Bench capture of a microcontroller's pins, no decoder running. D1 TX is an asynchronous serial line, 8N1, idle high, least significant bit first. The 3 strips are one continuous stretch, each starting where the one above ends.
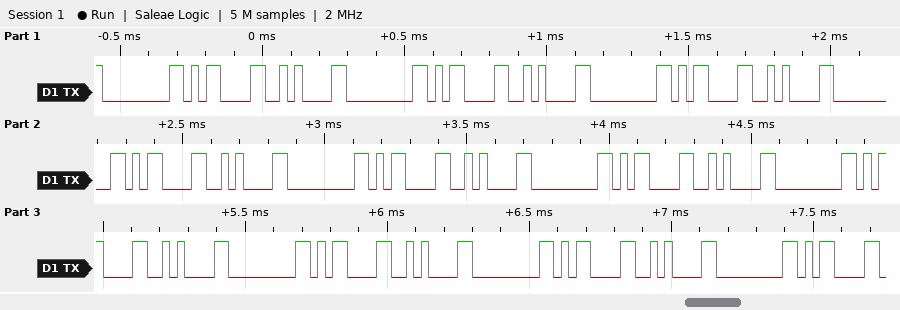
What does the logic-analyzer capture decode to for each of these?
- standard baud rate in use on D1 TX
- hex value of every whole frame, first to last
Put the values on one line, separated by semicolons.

38400 baud; 00 0D 0A 00 0D 0A 00 0D 0A 00 0D 0A 00 0D 0A 00 0D 0A 00 0D 0A 00 0D 0A 00 0D 0A 00 0D
